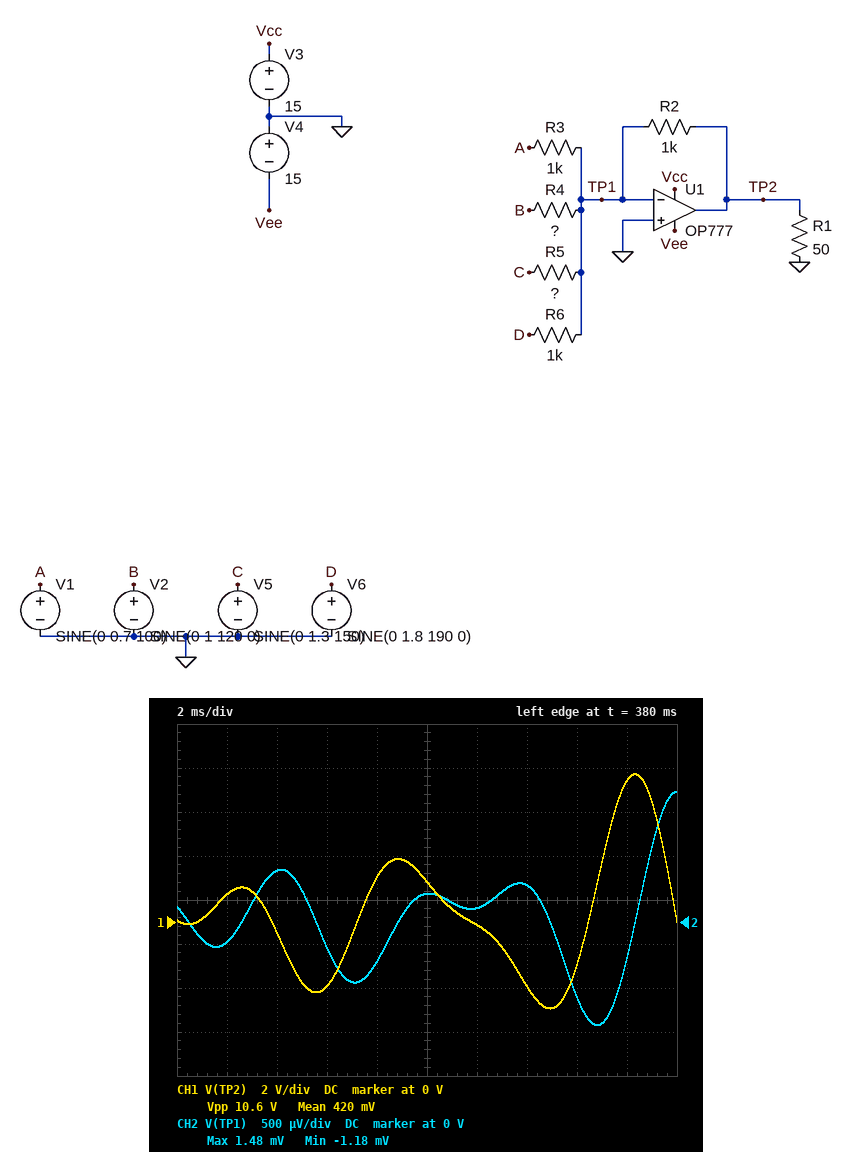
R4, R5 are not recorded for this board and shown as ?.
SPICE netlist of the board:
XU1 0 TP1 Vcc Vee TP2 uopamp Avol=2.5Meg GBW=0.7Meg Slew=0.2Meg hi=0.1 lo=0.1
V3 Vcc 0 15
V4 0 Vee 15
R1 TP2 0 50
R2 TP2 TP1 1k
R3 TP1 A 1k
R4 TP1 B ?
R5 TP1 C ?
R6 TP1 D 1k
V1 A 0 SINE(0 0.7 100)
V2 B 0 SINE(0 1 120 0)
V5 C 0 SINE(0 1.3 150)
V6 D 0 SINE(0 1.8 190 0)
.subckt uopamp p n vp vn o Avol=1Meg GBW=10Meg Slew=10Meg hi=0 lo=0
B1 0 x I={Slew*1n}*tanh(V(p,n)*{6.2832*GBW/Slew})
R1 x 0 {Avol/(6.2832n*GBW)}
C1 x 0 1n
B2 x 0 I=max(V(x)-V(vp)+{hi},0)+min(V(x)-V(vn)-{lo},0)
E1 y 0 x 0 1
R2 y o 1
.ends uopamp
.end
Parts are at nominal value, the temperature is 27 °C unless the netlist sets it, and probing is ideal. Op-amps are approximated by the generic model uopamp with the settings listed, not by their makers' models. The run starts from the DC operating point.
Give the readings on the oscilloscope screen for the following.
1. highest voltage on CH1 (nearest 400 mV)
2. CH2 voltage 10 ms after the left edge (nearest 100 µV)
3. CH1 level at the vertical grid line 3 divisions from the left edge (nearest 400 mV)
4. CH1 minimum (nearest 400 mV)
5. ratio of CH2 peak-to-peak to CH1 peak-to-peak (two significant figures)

6.8 V
300 µV
-2.8 V
-4.0 V
0.00025
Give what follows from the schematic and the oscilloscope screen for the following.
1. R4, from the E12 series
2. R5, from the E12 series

330 Ω
820 Ω
